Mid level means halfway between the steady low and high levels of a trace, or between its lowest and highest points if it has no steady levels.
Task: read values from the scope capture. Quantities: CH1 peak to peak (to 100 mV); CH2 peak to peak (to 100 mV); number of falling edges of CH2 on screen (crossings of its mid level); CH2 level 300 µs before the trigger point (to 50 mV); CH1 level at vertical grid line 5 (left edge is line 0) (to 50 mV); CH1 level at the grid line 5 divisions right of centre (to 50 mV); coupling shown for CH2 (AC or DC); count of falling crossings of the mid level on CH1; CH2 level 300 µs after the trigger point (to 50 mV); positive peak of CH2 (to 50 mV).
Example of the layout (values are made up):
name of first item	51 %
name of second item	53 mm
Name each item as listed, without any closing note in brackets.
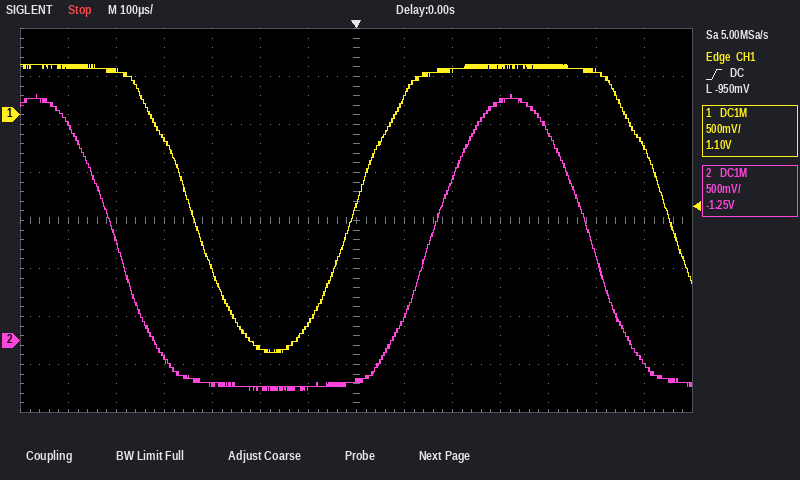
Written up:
CH1 peak to peak	3.00 V
CH2 peak to peak	3.10 V
number of falling edges of CH2 on screen	2
CH2 level 300 µs before the trigger point	-450 mV
CH1 level at vertical grid line 5 (left edge is line 0)	-2.40 V
CH1 level at the grid line 5 divisions right of centre	450 mV
coupling shown for CH2	DC
count of falling crossings of the mid level on CH1	2
CH2 level 300 µs after the trigger point	2.50 V
positive peak of CH2	2.55 V
